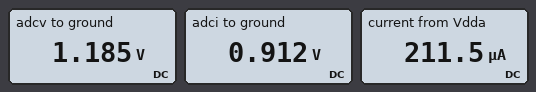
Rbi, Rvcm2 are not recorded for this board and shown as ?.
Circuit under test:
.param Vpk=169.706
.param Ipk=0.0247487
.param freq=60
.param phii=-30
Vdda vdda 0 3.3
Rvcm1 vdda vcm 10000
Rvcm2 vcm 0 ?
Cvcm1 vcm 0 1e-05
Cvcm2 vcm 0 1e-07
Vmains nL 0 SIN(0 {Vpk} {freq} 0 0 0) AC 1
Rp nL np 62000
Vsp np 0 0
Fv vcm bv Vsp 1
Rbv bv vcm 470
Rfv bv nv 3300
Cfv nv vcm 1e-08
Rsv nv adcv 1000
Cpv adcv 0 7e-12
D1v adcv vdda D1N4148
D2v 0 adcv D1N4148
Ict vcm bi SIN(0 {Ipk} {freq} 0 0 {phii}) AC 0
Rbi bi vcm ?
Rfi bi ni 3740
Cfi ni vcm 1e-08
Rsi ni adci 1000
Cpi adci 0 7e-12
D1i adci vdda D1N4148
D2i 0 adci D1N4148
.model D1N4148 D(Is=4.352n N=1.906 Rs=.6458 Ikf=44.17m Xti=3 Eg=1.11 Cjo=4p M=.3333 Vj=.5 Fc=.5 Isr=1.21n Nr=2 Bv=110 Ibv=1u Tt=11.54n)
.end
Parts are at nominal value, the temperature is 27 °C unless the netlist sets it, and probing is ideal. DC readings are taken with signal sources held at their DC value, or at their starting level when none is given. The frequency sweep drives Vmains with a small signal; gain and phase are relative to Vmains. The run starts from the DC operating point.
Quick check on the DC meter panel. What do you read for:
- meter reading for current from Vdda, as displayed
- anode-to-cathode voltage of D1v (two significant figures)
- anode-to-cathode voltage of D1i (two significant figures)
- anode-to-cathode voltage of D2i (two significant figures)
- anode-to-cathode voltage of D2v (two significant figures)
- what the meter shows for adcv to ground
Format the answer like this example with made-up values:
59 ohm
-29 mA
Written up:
211.5 µA
-2.1 V
-2.4 V
-910 mV
-1.2 V
1.185 V
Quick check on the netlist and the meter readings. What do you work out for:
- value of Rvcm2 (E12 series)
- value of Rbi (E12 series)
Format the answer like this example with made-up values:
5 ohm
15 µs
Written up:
5.6 kΩ
22 Ω
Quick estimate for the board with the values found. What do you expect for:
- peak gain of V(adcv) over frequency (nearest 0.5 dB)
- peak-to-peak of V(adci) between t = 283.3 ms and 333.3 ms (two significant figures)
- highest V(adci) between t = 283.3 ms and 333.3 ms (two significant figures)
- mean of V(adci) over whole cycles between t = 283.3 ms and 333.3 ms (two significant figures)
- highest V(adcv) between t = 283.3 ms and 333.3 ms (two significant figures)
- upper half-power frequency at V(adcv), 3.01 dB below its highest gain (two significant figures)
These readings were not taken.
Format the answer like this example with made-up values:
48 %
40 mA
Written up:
-42.5 dB
1.1 V
1.7 V
1.2 V
2.5 V
4.2 kHz
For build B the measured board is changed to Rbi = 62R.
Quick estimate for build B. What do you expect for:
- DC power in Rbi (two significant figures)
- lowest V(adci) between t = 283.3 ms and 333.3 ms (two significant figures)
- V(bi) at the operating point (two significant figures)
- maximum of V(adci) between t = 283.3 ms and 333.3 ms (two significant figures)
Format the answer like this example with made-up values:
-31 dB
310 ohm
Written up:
9.5 mW
-330 mV
420 mV
2.7 V
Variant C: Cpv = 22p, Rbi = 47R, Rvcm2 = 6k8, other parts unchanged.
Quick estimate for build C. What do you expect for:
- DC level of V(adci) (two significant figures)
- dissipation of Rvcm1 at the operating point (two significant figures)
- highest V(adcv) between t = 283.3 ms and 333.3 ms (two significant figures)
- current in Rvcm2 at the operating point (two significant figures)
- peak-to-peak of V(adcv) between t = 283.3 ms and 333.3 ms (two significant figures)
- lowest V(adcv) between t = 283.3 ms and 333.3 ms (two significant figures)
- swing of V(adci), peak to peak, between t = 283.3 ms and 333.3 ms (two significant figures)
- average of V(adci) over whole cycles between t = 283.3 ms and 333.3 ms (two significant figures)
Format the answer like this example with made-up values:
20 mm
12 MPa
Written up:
750 mV
390 µW
2.6 V
200 µA
2.6 V
49 mV
2.3 V
1.3 V
